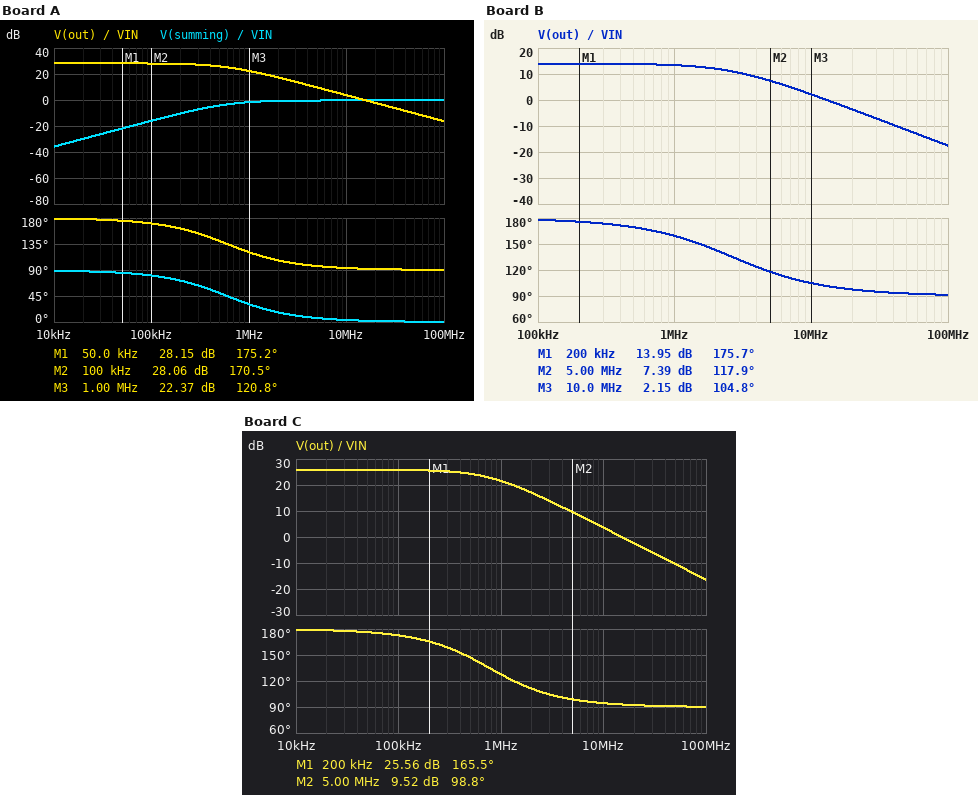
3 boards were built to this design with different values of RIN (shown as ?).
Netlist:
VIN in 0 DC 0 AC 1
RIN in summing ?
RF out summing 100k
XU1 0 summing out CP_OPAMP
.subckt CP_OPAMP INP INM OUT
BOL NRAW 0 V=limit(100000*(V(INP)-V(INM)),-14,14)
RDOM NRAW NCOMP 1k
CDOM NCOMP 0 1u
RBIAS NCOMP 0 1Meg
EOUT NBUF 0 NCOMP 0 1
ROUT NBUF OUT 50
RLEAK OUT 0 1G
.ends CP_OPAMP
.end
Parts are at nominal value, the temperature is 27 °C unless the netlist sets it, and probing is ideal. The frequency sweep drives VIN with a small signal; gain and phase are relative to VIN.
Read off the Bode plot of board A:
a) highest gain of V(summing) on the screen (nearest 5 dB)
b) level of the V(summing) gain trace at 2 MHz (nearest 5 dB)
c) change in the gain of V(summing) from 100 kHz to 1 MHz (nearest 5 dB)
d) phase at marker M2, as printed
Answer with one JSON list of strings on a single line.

["0 dB", "0 dB", "15 dB", "170.5 deg"]
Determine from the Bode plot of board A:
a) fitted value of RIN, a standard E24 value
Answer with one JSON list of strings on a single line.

["3.9 kΩ"]
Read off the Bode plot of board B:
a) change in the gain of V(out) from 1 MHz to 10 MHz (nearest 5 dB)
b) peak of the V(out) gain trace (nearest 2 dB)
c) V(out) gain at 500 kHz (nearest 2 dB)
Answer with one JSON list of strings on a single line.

["-10 dB", "14 dB", "14 dB"]
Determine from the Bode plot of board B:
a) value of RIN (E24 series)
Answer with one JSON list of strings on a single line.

["20 kΩ"]
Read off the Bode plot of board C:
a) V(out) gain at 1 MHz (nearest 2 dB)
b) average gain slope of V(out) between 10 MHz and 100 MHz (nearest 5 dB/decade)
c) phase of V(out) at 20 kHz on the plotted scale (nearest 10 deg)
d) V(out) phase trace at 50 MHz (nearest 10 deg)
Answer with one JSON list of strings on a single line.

["22 dB", "-20 dB/decade", "180 deg", "90 deg"]
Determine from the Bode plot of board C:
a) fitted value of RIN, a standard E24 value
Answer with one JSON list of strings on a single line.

["5.1 kΩ"]
